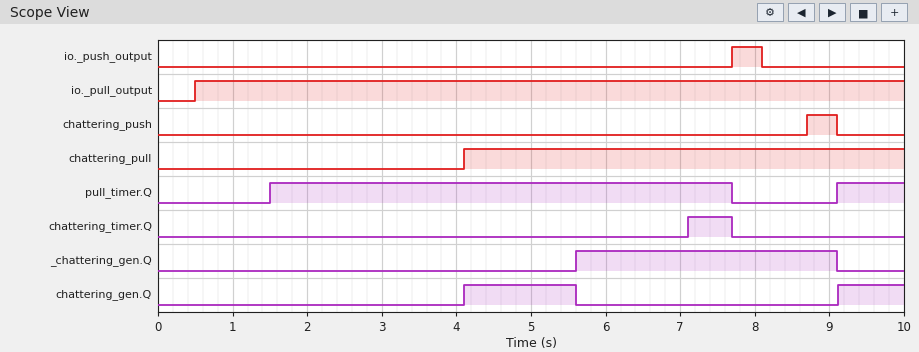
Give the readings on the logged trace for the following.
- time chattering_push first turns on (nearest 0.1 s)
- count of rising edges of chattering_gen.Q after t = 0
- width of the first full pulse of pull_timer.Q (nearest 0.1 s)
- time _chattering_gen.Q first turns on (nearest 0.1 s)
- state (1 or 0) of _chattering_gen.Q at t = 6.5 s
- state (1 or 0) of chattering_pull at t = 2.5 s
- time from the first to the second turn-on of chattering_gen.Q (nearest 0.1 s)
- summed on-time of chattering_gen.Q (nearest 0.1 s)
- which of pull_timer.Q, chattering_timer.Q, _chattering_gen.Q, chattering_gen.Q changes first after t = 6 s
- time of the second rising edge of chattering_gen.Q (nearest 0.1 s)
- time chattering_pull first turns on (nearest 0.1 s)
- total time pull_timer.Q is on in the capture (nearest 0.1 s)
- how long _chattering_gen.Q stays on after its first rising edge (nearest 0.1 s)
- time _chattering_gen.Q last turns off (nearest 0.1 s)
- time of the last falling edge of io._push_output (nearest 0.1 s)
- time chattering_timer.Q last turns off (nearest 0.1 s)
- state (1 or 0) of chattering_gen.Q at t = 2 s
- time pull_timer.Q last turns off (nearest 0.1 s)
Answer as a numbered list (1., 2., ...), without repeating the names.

1. 8.7 s
2. 2
3. 6.2 s
4. 5.6 s
5. 1
6. 0
7. 5.0 s
8. 2.4 s
9. chattering_timer.Q
10. 9.1 s
11. 4.1 s
12. 7.1 s
13. 3.5 s
14. 9.1 s
15. 8.1 s
16. 7.7 s
17. 0
18. 7.7 s
